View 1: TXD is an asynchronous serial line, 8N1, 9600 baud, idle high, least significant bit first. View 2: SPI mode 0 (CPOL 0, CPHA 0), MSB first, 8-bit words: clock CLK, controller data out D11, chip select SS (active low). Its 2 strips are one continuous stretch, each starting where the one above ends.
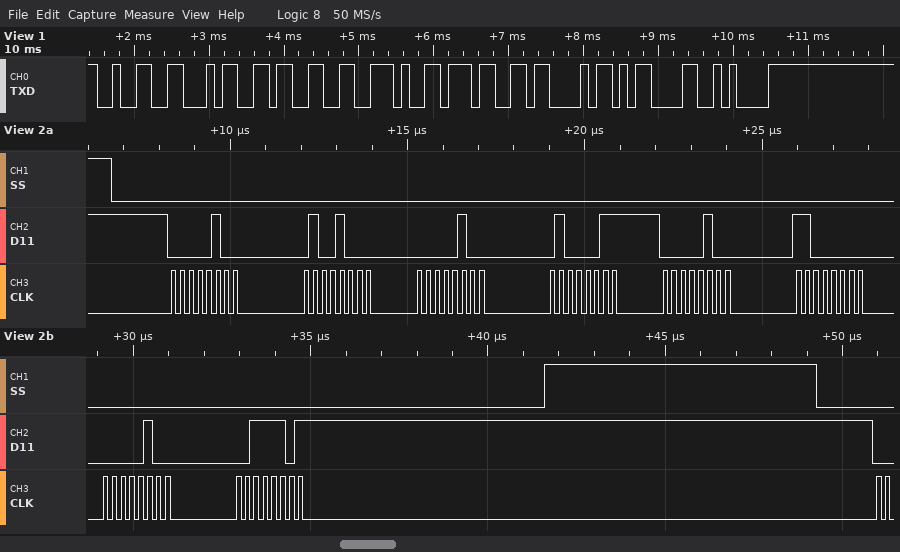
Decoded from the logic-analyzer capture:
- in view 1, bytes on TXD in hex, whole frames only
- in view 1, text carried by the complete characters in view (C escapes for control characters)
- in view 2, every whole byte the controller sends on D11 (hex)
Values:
0x32 0x34 0x33 0x2E 0x37 0x43 0x0D 0x0A
"243.7C\r\n"
04 48 04 43 04 C0 04 3D
